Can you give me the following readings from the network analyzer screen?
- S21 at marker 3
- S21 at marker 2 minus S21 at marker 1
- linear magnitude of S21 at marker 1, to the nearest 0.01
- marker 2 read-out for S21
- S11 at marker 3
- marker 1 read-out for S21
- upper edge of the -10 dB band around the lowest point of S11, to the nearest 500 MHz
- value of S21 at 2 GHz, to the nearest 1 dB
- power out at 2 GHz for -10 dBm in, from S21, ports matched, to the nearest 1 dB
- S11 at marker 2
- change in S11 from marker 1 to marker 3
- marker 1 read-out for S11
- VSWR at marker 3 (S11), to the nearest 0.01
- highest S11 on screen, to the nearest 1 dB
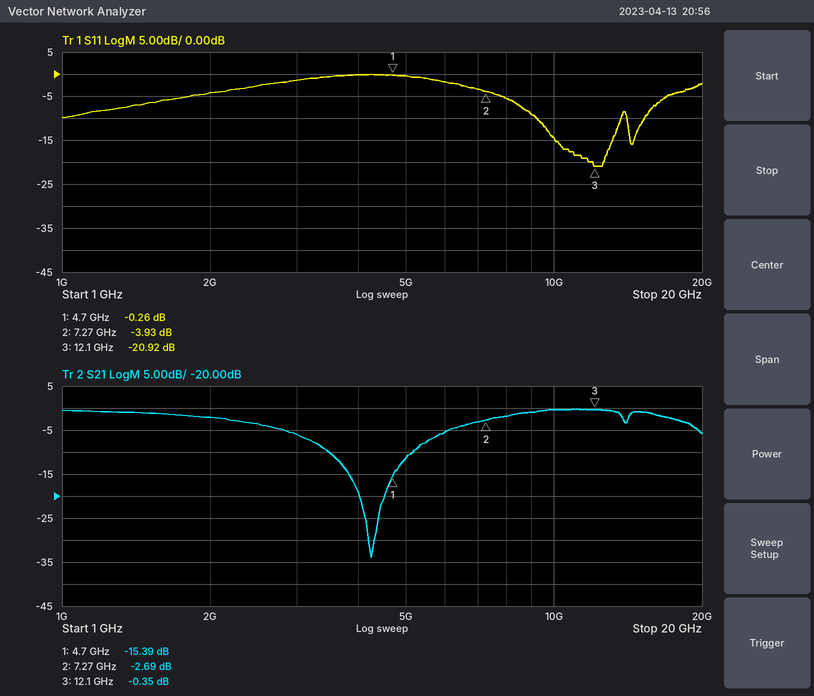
-0.35 dB
12.70 dB
0.17
-2.69 dB
-20.92 dB
-15.39 dB
13.5 GHz
-2 dB
-12 dBm
-3.93 dB
-20.66 dB
-0.26 dB
1.20
0 dB
